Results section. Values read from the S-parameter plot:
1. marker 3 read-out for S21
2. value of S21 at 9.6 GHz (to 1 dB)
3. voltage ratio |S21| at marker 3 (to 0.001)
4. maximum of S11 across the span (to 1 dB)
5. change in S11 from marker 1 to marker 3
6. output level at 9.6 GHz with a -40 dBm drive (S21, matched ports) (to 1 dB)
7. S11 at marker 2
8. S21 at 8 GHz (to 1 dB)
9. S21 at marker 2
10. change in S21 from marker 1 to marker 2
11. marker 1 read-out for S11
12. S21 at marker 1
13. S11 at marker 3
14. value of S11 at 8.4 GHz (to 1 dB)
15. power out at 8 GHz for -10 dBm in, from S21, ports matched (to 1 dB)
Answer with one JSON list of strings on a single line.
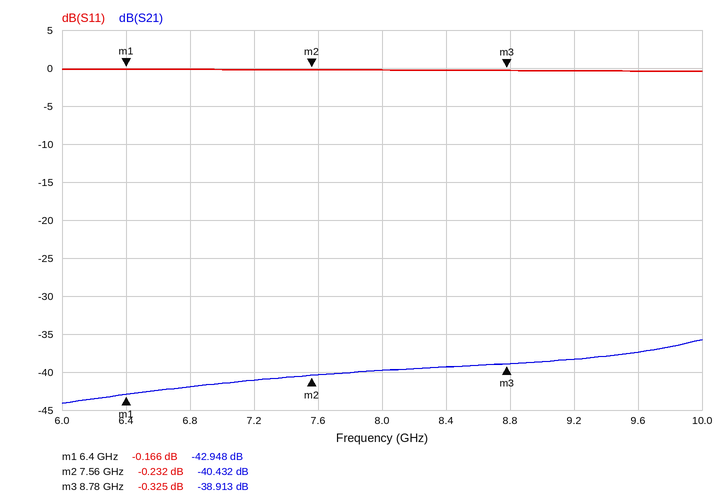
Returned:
["-38.913 dB", "-37 dB", "0.011", "0 dB", "-0.159 dB", "-77 dBm", "-0.232 dB", "-40 dB", "-40.432 dB", "2.516 dB", "-0.166 dB", "-42.948 dB", "-0.325 dB", "0 dB", "-50 dBm"]
